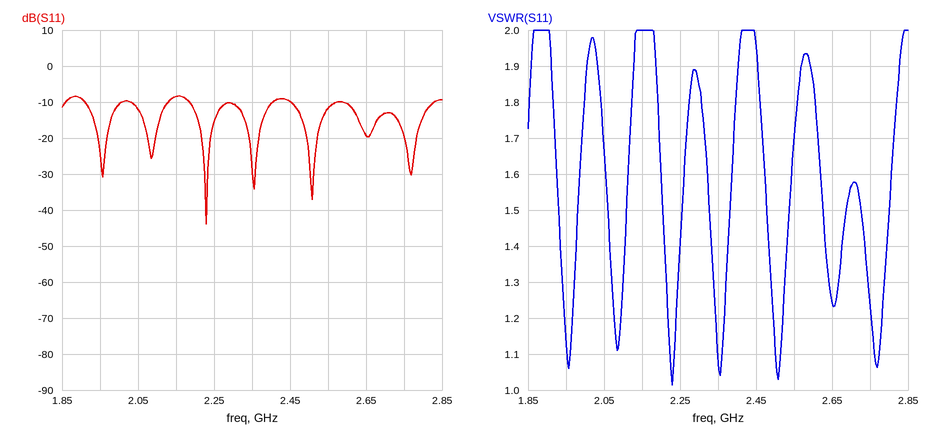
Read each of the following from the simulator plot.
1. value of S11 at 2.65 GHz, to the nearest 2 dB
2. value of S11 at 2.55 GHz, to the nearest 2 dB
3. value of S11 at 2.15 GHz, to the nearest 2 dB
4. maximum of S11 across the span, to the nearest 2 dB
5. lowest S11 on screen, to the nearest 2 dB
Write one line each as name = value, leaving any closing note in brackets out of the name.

value of S11 at 2.65 GHz, to the nearest 2 dB = -20 dB
value of S11 at 2.55 GHz, to the nearest 2 dB = -12 dB
value of S11 at 2.15 GHz, to the nearest 2 dB = -8 dB
maximum of S11 across the span, to the nearest 2 dB = -8 dB
lowest S11 on screen, to the nearest 2 dB = -44 dB
